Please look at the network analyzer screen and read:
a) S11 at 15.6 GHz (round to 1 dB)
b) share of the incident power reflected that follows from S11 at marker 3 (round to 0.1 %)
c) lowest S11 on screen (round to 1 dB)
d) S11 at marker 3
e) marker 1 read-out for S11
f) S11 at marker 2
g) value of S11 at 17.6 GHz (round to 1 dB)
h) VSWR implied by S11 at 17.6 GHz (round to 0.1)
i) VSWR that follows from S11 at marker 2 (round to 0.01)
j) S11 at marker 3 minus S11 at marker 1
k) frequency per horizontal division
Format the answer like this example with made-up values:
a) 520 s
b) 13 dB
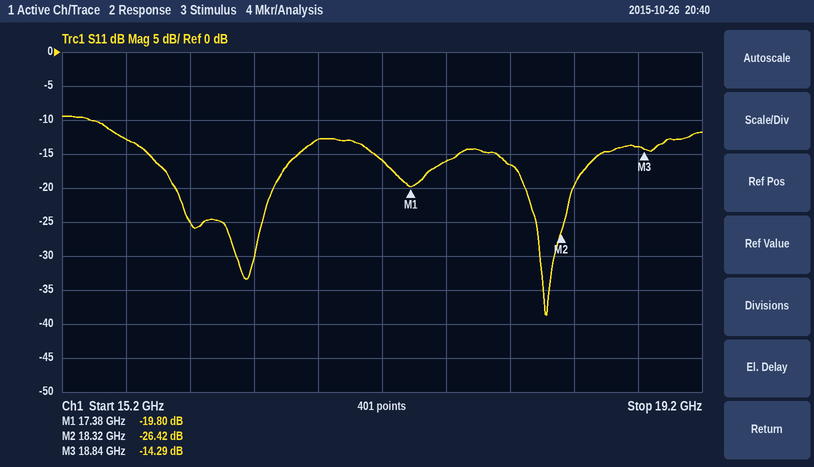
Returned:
a) -13 dB
b) 3.7 %
c) -39 dB
d) -14.29 dB
e) -19.80 dB
f) -26.42 dB
g) -16 dB
h) 1.4
i) 1.10
j) 5.51 dB
k) 400 MHz
